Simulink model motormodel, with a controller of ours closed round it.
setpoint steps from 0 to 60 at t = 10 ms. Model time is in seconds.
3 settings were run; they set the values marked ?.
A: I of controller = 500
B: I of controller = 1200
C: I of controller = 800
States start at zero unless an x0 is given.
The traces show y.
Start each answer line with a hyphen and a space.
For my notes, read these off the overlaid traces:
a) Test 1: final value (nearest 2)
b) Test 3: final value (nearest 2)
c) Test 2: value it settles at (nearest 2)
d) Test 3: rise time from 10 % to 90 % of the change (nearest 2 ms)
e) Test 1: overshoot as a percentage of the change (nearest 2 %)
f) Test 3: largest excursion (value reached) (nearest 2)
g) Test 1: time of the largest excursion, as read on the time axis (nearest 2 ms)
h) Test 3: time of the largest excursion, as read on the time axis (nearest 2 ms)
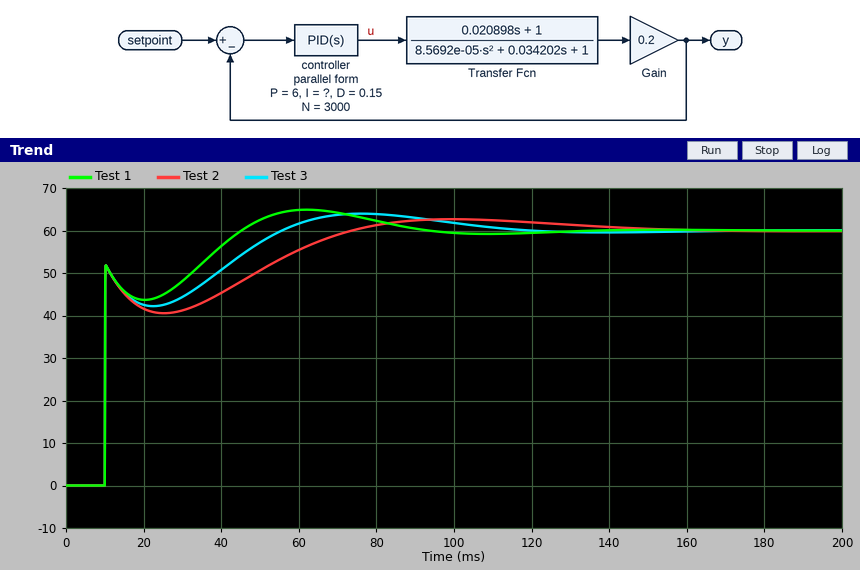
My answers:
- 60
- 60
- 60
- 34 ms
- 8 %
- 64
- 62 ms
- 76 ms
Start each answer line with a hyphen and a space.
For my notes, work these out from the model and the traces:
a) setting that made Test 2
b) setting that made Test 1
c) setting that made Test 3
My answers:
- A
- B
- C
